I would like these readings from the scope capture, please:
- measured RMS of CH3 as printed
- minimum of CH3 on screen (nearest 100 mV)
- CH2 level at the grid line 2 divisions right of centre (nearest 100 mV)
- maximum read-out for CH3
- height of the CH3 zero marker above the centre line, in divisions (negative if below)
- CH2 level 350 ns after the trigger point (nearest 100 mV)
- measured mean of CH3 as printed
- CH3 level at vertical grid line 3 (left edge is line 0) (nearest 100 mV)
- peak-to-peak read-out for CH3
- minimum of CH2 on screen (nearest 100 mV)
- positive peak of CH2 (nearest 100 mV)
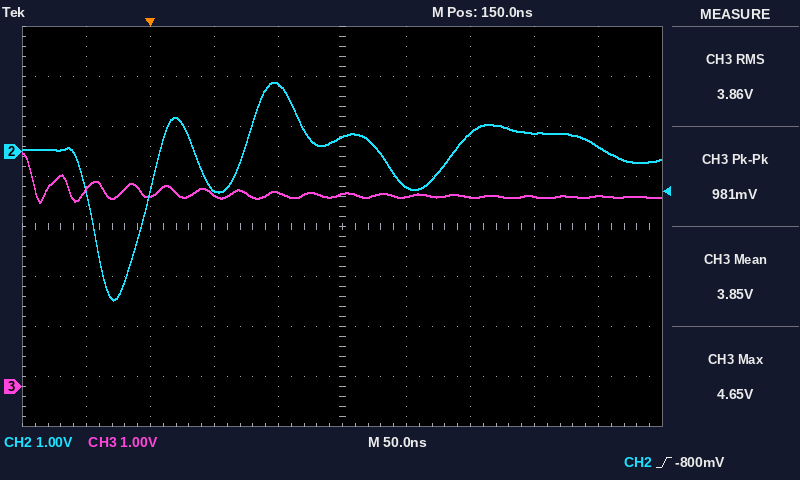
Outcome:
3.86 V
3.7 V
400 mV
4.65 V
-3.2 div
100 mV
3.85 V
3.8 V
981 mV
-3.0 V
1.4 V
